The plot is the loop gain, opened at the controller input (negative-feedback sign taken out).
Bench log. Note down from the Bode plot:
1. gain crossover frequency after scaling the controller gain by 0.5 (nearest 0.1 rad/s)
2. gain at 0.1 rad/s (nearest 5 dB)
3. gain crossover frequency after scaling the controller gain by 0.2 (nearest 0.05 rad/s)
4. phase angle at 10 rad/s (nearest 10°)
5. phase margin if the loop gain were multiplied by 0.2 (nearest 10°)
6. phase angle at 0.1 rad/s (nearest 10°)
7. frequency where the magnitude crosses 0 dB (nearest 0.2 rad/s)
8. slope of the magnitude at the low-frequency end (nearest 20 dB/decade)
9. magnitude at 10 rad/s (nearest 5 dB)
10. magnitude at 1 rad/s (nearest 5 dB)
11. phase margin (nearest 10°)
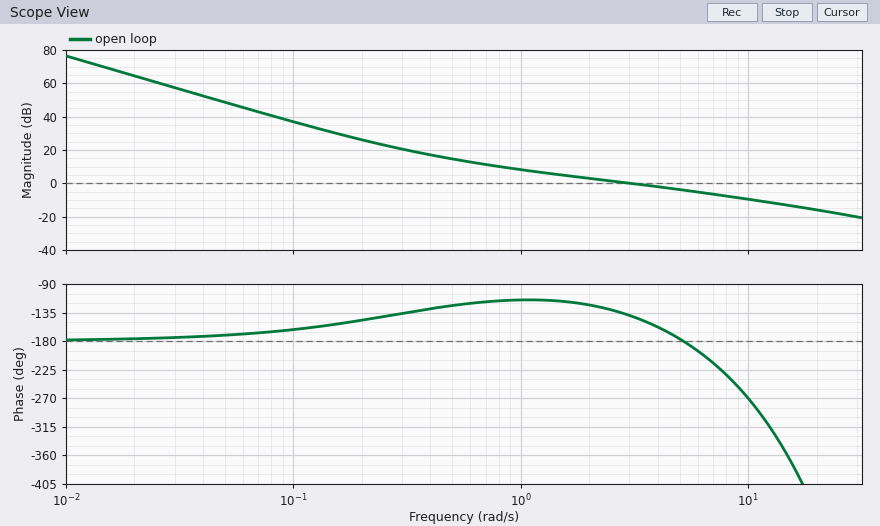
1.3 rad/s
35 dB
0.55 rad/s
-270°
60°
-160°
3.0 rad/s
-40 dB/decade
-10 dB
10 dB
40°
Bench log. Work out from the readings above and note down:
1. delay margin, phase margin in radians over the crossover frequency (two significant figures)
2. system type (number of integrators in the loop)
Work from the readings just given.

0.23 s
2
